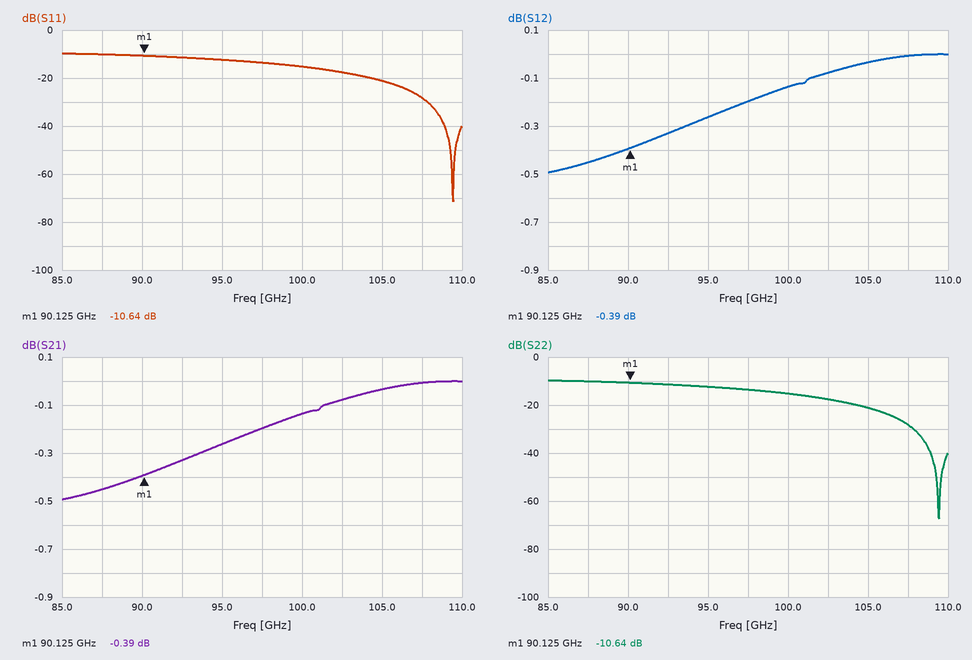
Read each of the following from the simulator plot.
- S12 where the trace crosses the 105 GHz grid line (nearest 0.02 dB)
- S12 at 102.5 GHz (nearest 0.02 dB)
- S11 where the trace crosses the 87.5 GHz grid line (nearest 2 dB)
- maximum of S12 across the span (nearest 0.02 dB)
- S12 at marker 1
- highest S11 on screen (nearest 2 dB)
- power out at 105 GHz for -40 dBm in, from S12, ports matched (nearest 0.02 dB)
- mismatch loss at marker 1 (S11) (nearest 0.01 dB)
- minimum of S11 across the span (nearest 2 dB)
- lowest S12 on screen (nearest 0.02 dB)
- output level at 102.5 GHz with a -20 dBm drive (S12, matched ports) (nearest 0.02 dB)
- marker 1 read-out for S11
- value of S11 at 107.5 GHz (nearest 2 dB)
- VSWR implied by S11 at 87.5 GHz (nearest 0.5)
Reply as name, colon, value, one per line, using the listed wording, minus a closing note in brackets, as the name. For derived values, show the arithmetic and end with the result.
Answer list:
S12 where the trace crosses the 105 GHz grid line: -0.04 dB
S12 at 102.5 GHz: -0.08 dB
S11 where the trace crosses the 87.5 GHz grid line: -10 dB
maximum of S12 across the span: 0.00 dB
S12 at marker 1: -0.39 dB
highest S11 on screen: -10 dB
power out at 105 GHz for -40 dBm in, from S12, ports matched: -40 dBm + (-0.04 dB) = -40.04 dBm
mismatch loss at marker 1 (S11): −10 log10(1 − 10^(-10.64/10)) ≈ 0.39 dB
minimum of S11 across the span: -72 dB
lowest S12 on screen: -0.50 dB
output level at 102.5 GHz with a -20 dBm drive (S12, matched ports): -20 dBm + (-0.08 dB) = -20.08 dBm
marker 1 read-out for S11: -10.64 dB
value of S11 at 107.5 GHz: -28 dB
VSWR implied by S11 at 87.5 GHz: |Γ| = 10^(-10/20) = 0.3162; VSWR = (1 + 0.3162)/(1 − 0.3162) ≈ 1.92, so 2.0 to the nearest 0.5
